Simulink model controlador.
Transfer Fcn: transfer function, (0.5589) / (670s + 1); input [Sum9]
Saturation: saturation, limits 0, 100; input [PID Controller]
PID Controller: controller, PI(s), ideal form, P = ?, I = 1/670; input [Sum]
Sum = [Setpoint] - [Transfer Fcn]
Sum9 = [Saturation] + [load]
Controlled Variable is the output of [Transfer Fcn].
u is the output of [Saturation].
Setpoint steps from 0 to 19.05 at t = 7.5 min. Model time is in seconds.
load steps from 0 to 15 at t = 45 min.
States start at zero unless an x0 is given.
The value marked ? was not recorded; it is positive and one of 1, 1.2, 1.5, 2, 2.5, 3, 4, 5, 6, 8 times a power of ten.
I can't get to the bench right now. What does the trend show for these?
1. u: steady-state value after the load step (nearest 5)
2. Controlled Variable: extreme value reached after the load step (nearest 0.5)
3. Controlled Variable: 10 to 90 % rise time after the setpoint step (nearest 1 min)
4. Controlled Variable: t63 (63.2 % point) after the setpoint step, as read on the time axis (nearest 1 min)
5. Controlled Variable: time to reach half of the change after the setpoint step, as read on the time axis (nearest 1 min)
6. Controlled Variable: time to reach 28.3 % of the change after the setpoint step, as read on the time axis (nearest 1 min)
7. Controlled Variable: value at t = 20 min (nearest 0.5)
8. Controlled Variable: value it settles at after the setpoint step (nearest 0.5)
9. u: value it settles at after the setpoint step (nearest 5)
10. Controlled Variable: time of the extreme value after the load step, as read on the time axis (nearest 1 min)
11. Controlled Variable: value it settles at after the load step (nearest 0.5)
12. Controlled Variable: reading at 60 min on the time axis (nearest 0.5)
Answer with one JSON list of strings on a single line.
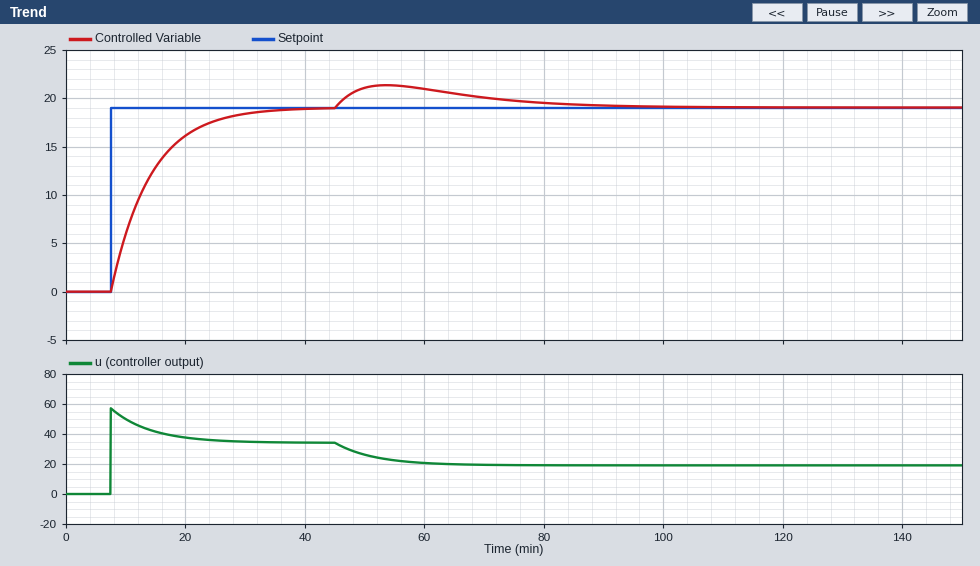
["20", "21.5", "15 min", "14 min", "12 min", "10 min", "16.0", "19.0", "35", "54 min", "19.0", "21.0"]
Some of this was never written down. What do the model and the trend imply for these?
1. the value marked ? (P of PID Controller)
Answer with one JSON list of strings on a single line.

["3"]
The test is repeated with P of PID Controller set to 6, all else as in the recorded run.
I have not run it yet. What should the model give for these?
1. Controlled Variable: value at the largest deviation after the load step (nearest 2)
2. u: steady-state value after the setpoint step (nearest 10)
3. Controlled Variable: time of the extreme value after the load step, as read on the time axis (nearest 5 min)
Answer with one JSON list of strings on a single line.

["20", "30", "50 min"]
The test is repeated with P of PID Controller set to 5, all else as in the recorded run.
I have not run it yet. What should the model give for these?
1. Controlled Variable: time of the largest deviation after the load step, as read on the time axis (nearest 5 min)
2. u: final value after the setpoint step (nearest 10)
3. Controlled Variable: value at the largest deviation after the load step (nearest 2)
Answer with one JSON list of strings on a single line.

["50 min", "30", "20"]
